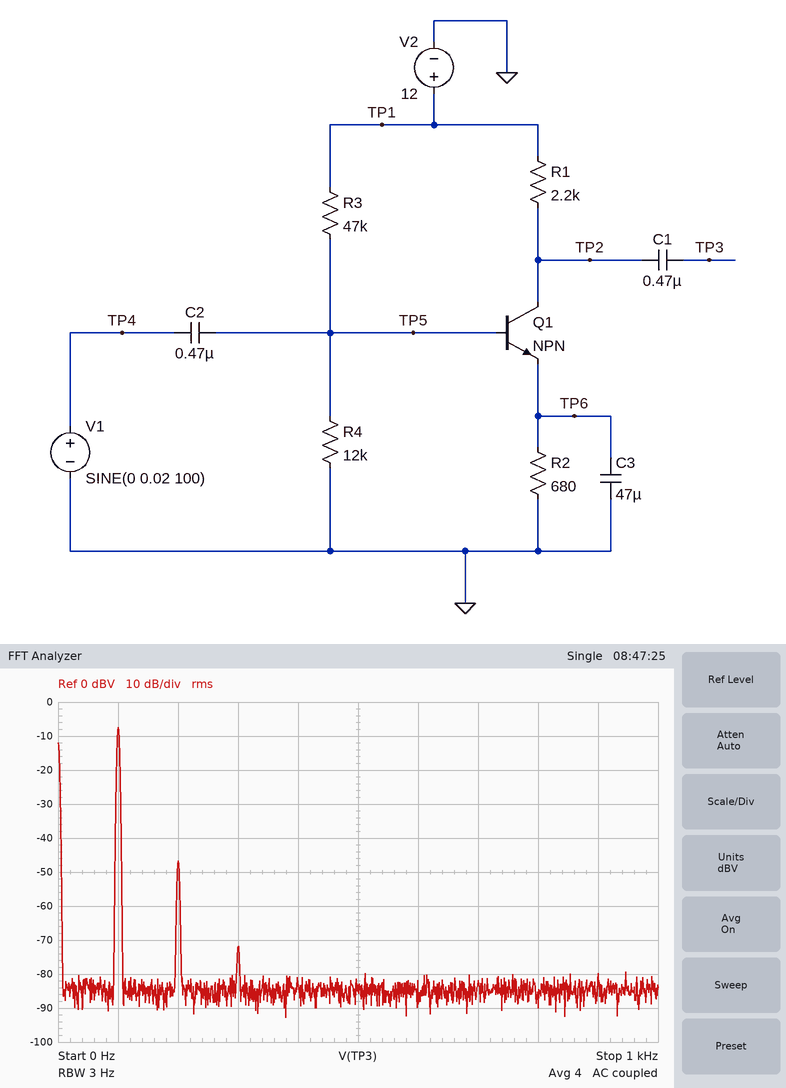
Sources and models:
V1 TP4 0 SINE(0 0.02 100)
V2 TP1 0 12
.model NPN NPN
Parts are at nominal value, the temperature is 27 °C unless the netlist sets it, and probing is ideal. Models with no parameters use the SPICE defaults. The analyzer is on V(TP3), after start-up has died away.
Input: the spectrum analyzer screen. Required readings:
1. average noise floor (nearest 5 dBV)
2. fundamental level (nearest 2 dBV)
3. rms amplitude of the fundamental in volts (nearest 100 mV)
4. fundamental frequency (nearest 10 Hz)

-85 dBV
-8 dBV
400 mV
100 Hz
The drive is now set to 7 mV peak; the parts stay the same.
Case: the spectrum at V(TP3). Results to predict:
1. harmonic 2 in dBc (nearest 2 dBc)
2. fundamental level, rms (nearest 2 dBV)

-48 dBc
-16 dBV
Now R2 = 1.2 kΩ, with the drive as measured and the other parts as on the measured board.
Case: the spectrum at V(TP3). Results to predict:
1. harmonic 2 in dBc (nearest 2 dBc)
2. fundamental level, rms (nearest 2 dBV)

-32 dBc
-8 dBV
